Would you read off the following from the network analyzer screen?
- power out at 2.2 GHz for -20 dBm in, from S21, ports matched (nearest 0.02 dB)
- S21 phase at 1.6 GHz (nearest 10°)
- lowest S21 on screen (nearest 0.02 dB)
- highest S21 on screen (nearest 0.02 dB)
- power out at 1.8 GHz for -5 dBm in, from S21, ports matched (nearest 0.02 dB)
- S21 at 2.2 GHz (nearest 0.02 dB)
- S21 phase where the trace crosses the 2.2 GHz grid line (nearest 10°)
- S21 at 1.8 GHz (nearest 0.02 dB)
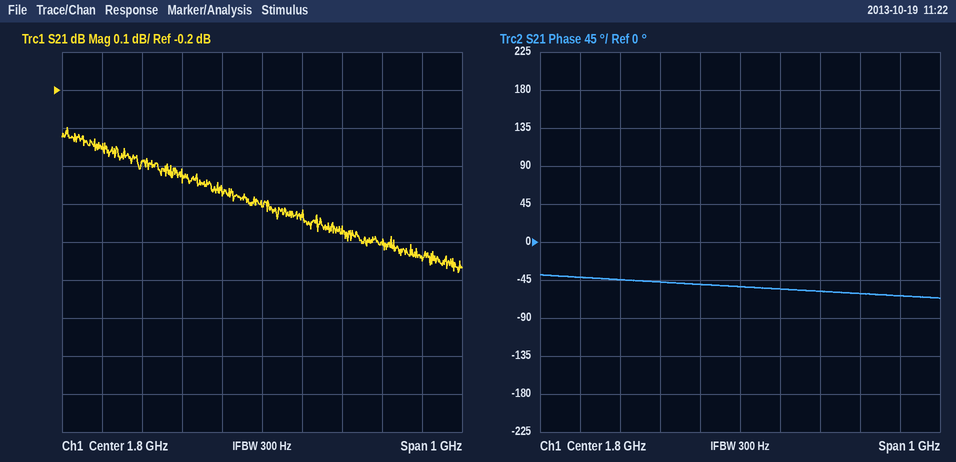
-20.64 dBm
-50°
-0.68 dB
-0.30 dB
-5.50 dBm
-0.64 dB
-60°
-0.50 dB
